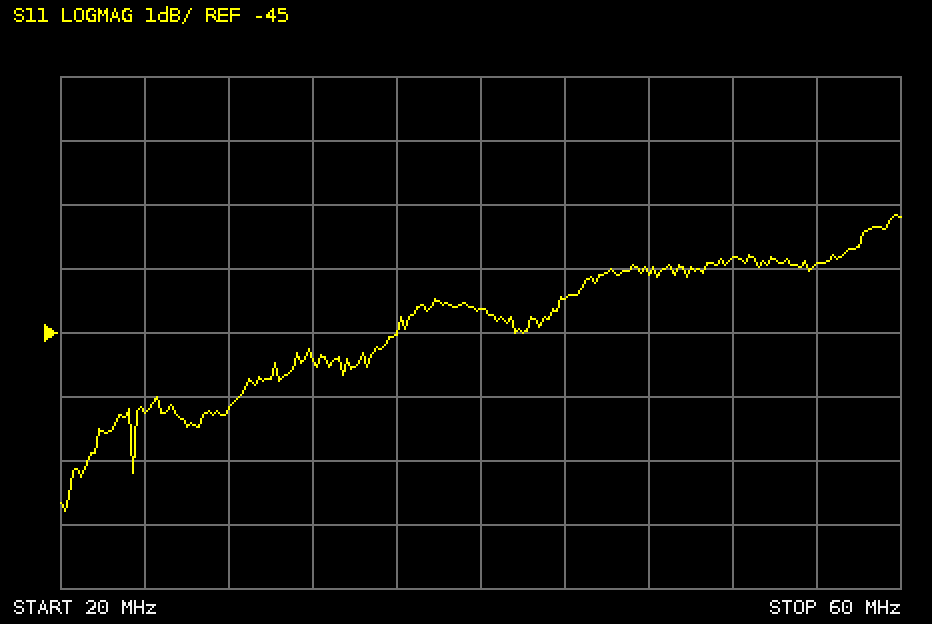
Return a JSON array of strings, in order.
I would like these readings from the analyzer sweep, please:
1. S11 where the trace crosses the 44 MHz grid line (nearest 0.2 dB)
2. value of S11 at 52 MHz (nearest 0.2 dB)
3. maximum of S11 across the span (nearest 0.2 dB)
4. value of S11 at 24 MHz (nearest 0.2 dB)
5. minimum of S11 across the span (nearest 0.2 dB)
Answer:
["-44.4 dB", "-43.8 dB", "-43.2 dB", "-46.2 dB", "-47.8 dB"]
